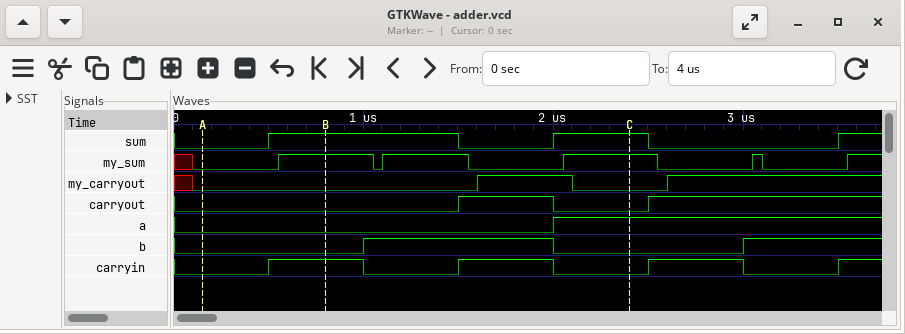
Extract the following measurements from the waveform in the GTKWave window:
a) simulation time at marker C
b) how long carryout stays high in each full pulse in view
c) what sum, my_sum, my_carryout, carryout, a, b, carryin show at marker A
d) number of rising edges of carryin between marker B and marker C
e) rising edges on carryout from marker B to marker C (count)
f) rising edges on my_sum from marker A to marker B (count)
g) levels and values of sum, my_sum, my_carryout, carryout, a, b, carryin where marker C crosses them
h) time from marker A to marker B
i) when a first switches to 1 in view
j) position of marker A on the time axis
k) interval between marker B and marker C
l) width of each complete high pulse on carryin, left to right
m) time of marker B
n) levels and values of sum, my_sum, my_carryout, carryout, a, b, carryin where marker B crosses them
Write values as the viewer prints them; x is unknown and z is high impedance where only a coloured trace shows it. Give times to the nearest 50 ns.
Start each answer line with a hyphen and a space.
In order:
- 2400 ns
- 500 ns
- sum=0, my_sum=0, my_carryout=0, carryout=0, a=0, b=0, carryin=0
- 1
- 1
- 1
- sum=1, my_sum=1, my_carryout=0, carryout=0, a=1, b=0, carryin=0
- 650 ns
- 2000 ns
- 150 ns
- 1600 ns
- 500 ns, 500 ns, 500 ns
- 800 ns
- sum=1, my_sum=1, my_carryout=0, carryout=0, a=0, b=0, carryin=1
